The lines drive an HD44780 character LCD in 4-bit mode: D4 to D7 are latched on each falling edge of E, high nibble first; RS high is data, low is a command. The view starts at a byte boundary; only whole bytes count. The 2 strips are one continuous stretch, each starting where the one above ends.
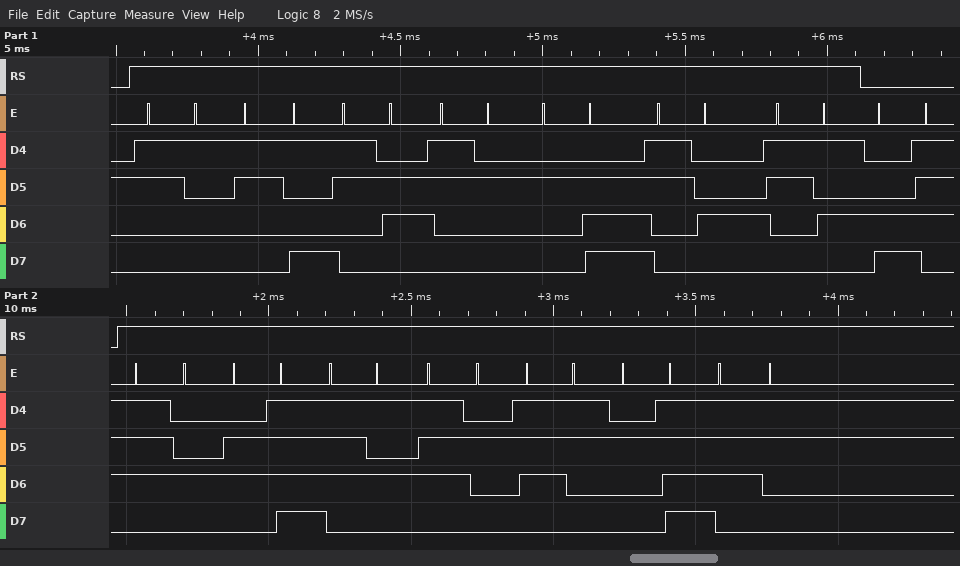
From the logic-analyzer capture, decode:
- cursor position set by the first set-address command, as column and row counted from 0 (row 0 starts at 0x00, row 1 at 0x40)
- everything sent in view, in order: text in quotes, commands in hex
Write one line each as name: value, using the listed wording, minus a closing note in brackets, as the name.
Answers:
cursor position set by the first set-address command, as column and row counted from 0: column 7, row 1
everything sent in view, in order: text in quotes, commands in hex: "1962.45" 0xC7 "tours/s"
